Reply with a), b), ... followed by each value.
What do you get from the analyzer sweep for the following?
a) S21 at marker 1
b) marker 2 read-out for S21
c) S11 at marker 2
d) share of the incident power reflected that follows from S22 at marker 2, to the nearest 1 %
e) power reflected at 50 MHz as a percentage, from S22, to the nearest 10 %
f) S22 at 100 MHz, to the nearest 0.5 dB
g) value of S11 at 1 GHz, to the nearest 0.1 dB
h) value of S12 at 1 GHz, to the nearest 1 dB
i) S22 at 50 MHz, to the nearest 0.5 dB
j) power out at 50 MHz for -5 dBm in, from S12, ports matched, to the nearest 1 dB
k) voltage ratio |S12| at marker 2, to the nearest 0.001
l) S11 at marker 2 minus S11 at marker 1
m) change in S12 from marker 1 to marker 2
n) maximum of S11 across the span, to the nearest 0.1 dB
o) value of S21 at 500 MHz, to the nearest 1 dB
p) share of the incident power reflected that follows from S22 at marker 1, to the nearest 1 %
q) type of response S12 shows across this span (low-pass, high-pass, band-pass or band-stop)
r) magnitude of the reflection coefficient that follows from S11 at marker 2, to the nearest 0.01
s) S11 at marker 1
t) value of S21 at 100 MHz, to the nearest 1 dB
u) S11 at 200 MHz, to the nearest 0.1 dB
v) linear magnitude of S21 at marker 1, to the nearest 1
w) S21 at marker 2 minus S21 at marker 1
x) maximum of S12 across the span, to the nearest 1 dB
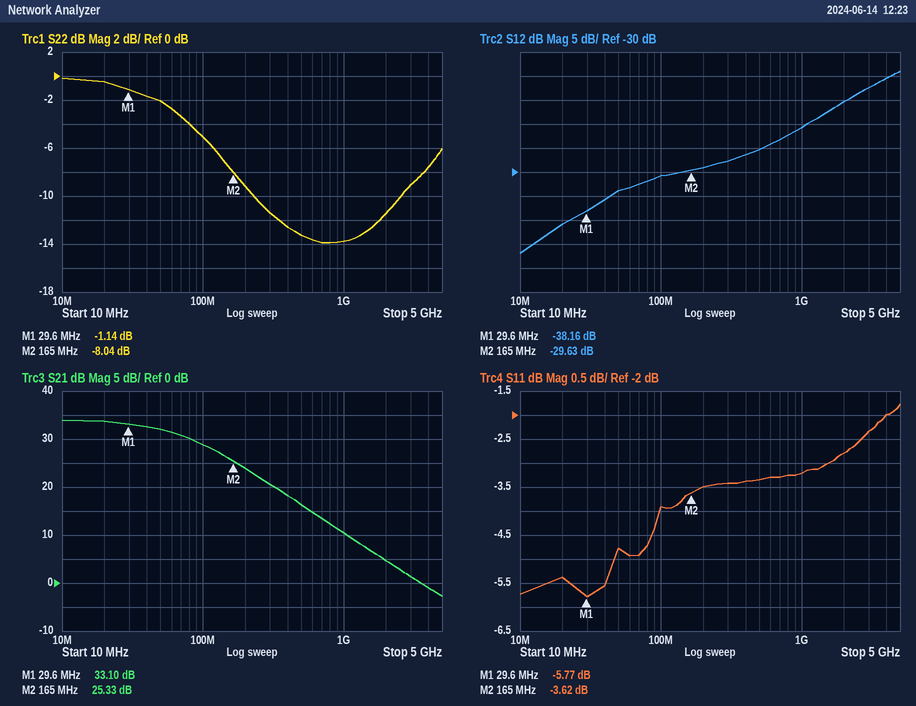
a) 33.10 dB
b) 25.33 dB
c) -3.62 dB
d) 16 %
e) 60 %
f) -5.0 dB
g) -3.2 dB
h) -21 dB
i) -2.0 dB
j) -39 dBm
k) 0.033
l) 2.15 dB
m) 8.53 dB
n) -1.8 dB
o) 16 dB
p) 77 %
q) high-pass
r) 0.66
s) -5.77 dB
t) 29 dB
u) -3.5 dB
v) 45
w) -7.77 dB
x) -9 dB
